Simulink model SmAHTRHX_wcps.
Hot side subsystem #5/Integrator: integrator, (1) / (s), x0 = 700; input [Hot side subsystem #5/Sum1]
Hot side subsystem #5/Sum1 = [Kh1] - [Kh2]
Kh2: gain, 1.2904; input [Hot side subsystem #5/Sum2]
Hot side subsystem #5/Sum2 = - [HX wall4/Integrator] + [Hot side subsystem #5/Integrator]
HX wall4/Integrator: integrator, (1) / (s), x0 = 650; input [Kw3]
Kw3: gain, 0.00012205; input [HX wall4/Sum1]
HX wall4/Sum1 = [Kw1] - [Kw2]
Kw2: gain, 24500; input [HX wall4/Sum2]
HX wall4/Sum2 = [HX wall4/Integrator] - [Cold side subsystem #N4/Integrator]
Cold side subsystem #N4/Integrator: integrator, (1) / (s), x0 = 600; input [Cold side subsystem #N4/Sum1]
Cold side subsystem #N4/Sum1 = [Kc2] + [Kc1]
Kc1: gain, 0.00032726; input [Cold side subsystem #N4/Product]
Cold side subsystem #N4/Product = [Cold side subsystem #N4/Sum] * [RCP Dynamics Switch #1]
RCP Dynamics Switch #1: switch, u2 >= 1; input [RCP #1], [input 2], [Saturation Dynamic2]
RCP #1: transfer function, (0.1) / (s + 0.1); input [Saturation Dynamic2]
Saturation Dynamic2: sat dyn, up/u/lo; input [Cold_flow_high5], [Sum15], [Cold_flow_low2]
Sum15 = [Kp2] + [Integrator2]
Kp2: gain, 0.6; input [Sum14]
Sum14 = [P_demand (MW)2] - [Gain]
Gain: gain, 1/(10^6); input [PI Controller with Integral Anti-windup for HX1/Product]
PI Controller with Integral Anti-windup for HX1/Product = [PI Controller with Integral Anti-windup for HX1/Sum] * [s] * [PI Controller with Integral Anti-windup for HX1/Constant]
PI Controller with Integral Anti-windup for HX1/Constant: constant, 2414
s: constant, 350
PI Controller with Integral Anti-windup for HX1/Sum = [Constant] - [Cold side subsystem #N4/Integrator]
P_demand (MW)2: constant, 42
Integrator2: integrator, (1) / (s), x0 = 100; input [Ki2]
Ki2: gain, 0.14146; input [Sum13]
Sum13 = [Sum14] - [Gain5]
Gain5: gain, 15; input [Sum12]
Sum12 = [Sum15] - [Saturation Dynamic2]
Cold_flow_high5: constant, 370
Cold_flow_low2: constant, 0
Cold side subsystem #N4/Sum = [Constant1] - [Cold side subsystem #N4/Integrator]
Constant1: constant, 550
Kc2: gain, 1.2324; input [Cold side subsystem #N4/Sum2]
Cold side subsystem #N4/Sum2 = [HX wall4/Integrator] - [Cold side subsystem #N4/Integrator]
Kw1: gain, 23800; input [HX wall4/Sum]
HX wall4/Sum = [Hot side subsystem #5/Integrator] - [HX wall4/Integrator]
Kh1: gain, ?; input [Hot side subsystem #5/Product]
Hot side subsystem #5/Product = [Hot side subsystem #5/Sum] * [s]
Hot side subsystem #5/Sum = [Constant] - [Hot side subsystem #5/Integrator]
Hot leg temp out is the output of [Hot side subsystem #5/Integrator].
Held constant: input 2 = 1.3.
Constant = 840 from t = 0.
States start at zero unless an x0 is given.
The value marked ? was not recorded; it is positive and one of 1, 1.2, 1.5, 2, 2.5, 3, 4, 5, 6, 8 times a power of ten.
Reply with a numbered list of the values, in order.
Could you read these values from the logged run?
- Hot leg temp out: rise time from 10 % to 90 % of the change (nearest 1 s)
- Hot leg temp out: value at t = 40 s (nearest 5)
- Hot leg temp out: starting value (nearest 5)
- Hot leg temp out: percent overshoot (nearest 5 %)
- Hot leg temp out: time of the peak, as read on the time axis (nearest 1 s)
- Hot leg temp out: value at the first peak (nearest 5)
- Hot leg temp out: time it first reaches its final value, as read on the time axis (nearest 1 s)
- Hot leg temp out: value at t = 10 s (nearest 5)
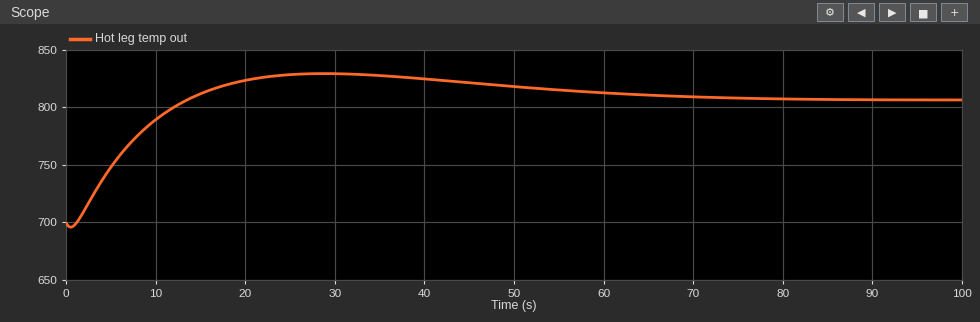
1. 9 s
2. 825
3. 700
4. 20 %
5. 29 s
6. 830
7. 14 s
8. 790
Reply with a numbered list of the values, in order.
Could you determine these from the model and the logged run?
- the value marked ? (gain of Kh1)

1. 0.001
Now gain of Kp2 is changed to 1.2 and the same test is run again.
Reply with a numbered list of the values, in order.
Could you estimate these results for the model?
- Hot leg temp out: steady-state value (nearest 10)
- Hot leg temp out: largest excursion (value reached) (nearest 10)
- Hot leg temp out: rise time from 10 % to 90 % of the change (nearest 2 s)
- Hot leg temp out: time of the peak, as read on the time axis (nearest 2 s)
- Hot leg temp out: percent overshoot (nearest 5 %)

1. 810
2. 820
3. 10 s
4. 26 s
5. 10 %
